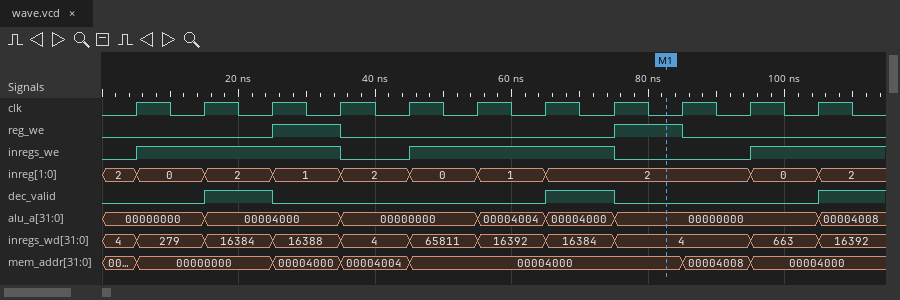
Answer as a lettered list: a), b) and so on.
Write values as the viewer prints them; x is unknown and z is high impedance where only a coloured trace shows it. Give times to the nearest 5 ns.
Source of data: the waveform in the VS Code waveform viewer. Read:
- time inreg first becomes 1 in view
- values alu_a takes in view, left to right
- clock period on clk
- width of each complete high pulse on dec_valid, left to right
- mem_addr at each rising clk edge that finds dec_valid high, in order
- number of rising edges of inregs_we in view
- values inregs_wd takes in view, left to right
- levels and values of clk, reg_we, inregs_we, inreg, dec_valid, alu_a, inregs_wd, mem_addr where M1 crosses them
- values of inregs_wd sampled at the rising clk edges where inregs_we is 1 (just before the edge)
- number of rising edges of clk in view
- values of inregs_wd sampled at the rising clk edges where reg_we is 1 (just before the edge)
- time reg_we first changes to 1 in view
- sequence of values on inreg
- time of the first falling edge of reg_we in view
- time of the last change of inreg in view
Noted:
a) 25 ns
b) 00000000, 00004000, 00000000, 00004004, 00004000, 00000000, 00004008
c) 10 ns
d) 10 ns, 10 ns
e) 00000000, 00004000
f) 3
g) 4, 279, 16384, 16388, 4, 65811, 16392, 16384, 4, 663, 16392
h) clk=0, reg_we=1, inregs_we=0, inreg=2, dec_valid=0, alu_a=00000000, inregs_wd=4, mem_addr=00004000
i) 279, 16384, 16388, 65811, 16392, 16384, 663
j) 11
k) 16388, 4
l) 25 ns
m) 2, 0, 2, 1, 2, 0, 1, 2, 0, 2
n) 35 ns
o) 105 ns
